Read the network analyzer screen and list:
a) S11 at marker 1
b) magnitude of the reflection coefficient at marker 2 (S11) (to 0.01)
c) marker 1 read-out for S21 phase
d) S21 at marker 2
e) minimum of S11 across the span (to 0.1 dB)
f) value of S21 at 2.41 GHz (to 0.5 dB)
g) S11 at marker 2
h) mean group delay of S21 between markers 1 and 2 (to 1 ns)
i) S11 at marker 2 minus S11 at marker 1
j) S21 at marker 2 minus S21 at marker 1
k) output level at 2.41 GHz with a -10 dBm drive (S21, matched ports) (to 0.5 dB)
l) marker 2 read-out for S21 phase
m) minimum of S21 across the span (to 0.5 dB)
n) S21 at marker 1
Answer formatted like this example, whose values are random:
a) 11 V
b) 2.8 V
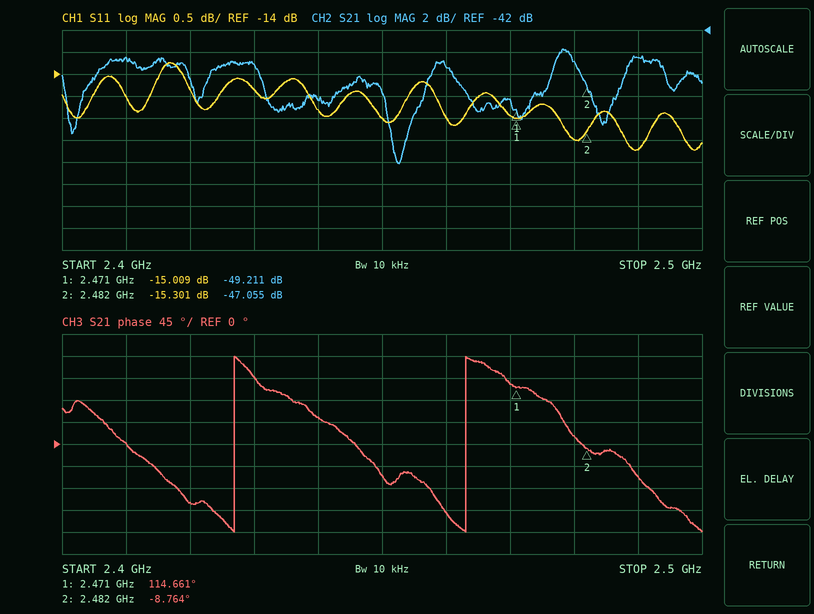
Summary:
a) -15.009 dB
b) 0.17
c) 114.661°
d) -47.055 dB
e) -15.7 dB
f) -44.5 dB
g) -15.301 dB
h) 31 ns
i) -0.292 dB
j) 2.156 dB
k) -54.5 dBm
l) -8.764°
m) -54.0 dB
n) -49.211 dB
